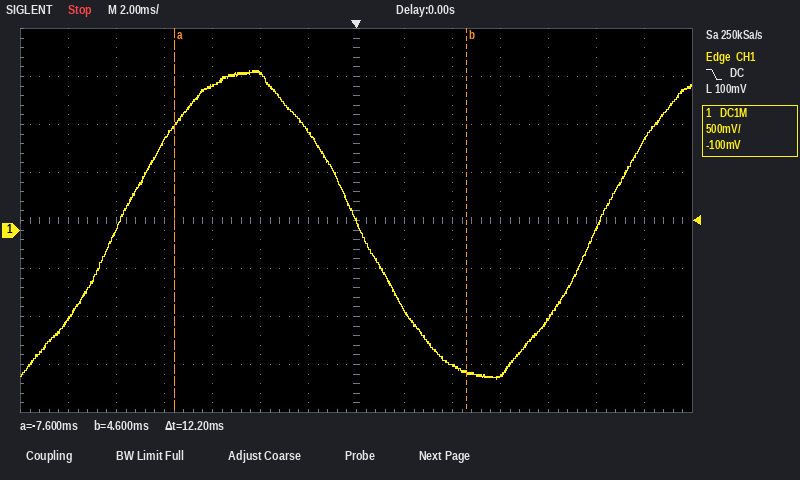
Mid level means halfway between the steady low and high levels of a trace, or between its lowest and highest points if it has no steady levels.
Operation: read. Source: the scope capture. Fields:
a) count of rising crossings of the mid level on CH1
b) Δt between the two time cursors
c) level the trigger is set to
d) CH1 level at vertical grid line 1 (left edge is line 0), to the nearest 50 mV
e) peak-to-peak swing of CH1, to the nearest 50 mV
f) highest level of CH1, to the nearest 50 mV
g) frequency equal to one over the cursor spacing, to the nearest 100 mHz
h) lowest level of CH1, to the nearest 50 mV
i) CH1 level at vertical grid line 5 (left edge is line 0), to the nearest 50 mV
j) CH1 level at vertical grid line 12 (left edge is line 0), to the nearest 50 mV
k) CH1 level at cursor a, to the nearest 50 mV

2
12.2 ms
100 mV
-950 mV
3.20 V
1.65 V
82.0 Hz
-1.55 V
1.65 V
0 mV
1.10 V
